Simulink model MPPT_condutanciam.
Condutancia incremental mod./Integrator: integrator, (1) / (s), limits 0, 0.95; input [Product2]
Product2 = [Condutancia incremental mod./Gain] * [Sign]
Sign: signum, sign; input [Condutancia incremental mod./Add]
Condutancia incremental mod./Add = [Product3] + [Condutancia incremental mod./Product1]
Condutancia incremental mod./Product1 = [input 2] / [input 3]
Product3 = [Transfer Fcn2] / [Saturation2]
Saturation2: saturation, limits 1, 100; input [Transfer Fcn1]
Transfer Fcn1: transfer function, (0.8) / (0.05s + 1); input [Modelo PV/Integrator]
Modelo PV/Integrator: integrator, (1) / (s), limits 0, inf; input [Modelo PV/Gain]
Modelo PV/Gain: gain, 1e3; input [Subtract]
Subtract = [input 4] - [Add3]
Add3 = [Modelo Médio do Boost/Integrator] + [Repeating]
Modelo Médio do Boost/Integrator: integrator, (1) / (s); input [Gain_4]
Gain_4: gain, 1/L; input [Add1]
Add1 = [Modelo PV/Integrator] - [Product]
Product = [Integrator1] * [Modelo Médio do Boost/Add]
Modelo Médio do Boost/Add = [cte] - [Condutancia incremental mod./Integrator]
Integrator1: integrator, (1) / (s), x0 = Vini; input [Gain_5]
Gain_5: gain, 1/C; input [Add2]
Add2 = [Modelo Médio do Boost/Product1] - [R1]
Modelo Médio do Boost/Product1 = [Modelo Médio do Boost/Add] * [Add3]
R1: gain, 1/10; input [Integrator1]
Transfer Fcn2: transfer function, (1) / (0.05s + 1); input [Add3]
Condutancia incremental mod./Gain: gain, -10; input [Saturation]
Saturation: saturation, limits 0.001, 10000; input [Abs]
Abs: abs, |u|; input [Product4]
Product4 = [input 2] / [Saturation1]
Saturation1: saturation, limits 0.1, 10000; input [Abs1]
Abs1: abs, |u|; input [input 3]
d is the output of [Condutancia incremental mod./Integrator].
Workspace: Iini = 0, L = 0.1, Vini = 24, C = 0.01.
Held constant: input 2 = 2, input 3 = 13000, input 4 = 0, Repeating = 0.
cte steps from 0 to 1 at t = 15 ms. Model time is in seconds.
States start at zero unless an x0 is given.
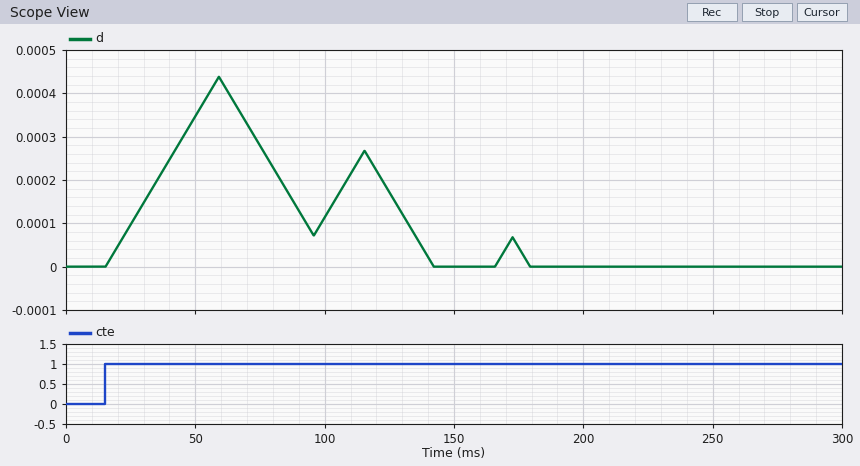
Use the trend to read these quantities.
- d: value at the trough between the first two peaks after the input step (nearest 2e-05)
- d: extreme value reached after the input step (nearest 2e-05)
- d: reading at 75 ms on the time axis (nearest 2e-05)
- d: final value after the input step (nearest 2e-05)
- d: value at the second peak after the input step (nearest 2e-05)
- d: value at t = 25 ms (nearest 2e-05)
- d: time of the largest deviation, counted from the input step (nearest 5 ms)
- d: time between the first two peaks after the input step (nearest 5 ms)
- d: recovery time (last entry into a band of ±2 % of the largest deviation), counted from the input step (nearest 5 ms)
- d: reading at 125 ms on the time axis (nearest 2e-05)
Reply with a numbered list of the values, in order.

1. 0.00008
2. 0.00044
3. 0.00028
4. 0.00000
5. 0.00026
6. 0.00010
7. 45 ms
8. 55 ms
9. 165 ms
10. 0.00018
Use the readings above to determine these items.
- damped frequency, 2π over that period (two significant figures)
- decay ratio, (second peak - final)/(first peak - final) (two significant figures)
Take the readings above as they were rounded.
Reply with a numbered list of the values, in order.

1. 0.11 rad/ms
2. 0.59
